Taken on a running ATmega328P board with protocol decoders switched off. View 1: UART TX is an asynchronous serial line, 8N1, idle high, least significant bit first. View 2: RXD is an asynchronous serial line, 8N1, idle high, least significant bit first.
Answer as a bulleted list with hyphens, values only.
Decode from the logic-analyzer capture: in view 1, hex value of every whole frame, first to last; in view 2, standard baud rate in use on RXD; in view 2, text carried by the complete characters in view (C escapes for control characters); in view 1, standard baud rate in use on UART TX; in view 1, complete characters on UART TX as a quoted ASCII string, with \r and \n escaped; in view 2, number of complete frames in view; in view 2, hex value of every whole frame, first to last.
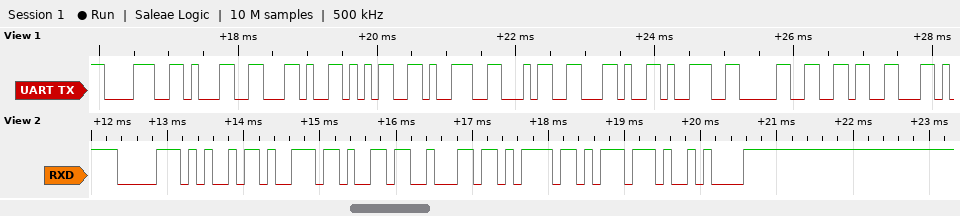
- 38 31 2C 35 39 34 2C 39 30 36
- 9600 baud
- "pin6low\n"
- 9600 baud
- "81,594,906"
- 8
- 70 69 6E 36 6C 6F 77 0A
